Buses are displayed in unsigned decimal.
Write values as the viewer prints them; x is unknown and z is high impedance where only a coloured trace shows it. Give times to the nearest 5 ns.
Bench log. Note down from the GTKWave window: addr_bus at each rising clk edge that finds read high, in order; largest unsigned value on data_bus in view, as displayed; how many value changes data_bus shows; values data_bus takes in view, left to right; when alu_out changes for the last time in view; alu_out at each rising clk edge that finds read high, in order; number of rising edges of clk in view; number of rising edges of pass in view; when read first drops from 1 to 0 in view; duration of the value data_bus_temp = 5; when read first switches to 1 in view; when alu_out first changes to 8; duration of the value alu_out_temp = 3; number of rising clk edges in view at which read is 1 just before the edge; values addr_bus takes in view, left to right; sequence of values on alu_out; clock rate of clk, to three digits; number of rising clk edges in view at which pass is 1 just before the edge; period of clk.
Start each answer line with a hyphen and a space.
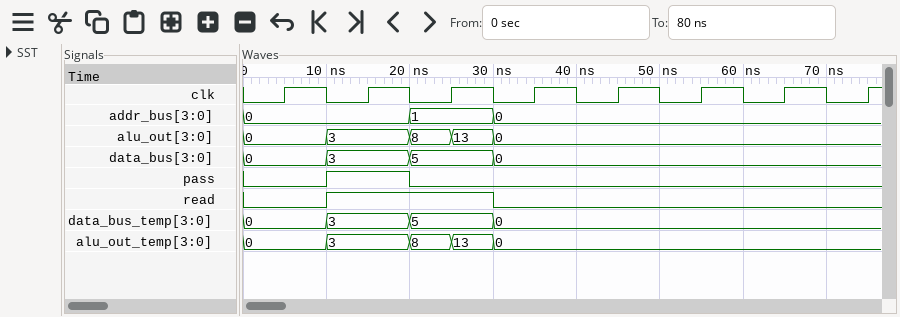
- 0, 1
- 5
- 3
- 0, 3, 5, 0
- 30 ns
- 3, 8
- 8
- 1
- 30 ns
- 10 ns
- 10 ns
- 20 ns
- 10 ns
- 2
- 0, 1, 0
- 0, 3, 8, 13, 0
- 100 MHz
- 1
- 10 ns
